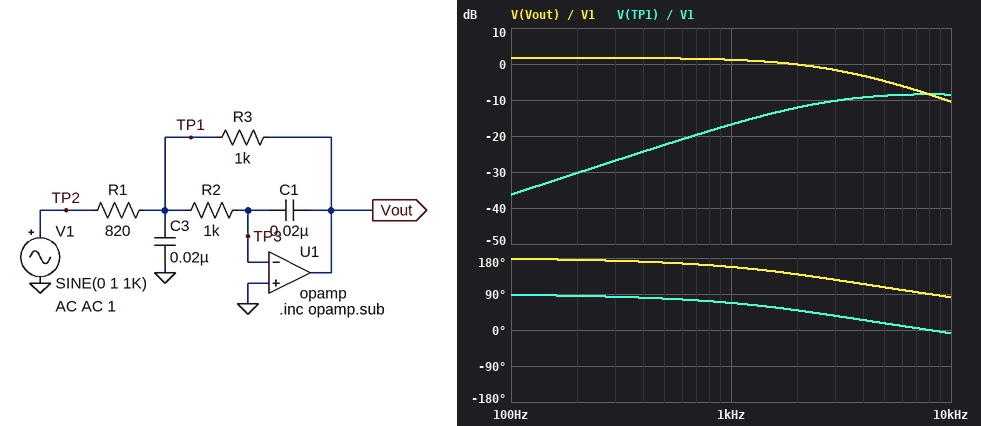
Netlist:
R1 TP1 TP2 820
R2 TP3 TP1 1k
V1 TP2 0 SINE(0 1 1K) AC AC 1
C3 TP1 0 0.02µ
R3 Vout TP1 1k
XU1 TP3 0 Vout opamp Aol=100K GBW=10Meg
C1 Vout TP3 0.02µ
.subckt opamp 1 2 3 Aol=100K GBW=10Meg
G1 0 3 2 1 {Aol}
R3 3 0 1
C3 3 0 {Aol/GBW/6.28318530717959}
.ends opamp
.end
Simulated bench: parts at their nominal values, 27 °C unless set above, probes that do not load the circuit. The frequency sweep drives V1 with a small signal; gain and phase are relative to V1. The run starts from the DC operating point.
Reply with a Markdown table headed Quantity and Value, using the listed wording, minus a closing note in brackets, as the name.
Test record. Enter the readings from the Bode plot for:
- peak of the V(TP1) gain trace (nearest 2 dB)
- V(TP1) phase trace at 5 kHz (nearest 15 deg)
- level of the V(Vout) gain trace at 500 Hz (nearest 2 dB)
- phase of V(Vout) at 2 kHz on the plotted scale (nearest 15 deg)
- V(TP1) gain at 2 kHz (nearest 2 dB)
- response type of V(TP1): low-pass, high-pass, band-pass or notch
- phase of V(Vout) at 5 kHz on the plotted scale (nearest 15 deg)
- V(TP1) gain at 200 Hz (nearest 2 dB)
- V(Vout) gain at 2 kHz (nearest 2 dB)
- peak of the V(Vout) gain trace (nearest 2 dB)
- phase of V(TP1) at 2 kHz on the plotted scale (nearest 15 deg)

| Quantity | Value |
|---|---|
| peak of the V(TP1) gain trace | -8 dB |
| V(TP1) phase trace at 5 kHz | 15 deg |
| level of the V(Vout) gain trace at 500 Hz | 2 dB |
| phase of V(Vout) at 2 kHz on the plotted scale | 135 deg |
| V(TP1) gain at 2 kHz | -12 dB |
| response type of V(TP1): low-pass, high-pass, band-pass or notch | high-pass |
| phase of V(Vout) at 5 kHz on the plotted scale | 105 deg |
| V(TP1) gain at 200 Hz | -30 dB |
| V(Vout) gain at 2 kHz | 0 dB |
| peak of the V(Vout) gain trace | 2 dB |
| phase of V(TP1) at 2 kHz on the plotted scale | 45 deg |
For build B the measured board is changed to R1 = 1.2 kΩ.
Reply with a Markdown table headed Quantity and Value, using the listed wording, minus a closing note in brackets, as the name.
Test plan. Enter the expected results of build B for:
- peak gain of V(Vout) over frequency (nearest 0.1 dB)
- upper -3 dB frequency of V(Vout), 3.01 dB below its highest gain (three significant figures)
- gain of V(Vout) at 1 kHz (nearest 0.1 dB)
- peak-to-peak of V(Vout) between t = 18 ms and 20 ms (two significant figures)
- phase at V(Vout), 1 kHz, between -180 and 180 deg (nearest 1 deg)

| Quantity | Value |
|---|---|
| peak gain of V(Vout) over frequency | -1.6 dB |
| upper -3 dB frequency of V(Vout), 3.01 dB below its highest gain | 3.20 kHz |
| gain of V(Vout) at 1 kHz | -2.0 dB |
| peak-to-peak of V(Vout) between t = 18 ms and 20 ms | 1.6 V |
| phase at V(Vout), 1 kHz, between -180 and 180 deg | 160 deg |
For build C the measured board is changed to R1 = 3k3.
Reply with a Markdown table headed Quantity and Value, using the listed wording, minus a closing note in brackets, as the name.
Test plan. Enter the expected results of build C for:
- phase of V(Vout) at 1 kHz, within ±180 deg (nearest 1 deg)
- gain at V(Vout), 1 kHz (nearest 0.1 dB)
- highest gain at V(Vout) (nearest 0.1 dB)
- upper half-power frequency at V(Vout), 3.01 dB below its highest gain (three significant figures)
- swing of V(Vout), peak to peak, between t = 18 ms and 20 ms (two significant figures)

| Quantity | Value |
|---|---|
| phase of V(Vout) at 1 kHz, within ±180 deg | 164 deg |
| gain at V(Vout), 1 kHz | -10.6 dB |
| highest gain at V(Vout) | -10.4 dB |
| upper half-power frequency at V(Vout), 3.01 dB below its highest gain | 4.20 kHz |
| swing of V(Vout), peak to peak, between t = 18 ms and 20 ms | 590 mV |
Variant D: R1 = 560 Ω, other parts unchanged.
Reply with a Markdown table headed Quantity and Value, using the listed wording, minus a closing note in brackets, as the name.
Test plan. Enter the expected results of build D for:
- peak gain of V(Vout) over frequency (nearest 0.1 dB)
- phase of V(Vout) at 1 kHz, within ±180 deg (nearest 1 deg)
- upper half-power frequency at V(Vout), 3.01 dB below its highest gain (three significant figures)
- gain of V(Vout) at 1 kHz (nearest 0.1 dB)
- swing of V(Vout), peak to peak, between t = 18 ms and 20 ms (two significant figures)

| Quantity | Value |
|---|---|
| peak gain of V(Vout) over frequency | 5.0 dB |
| phase of V(Vout) at 1 kHz, within ±180 deg | 154 deg |
| upper half-power frequency at V(Vout), 3.01 dB below its highest gain | 2.26 kHz |
| gain of V(Vout) at 1 kHz | 4.3 dB |
| swing of V(Vout), peak to peak, between t = 18 ms and 20 ms | 3.3 V |
